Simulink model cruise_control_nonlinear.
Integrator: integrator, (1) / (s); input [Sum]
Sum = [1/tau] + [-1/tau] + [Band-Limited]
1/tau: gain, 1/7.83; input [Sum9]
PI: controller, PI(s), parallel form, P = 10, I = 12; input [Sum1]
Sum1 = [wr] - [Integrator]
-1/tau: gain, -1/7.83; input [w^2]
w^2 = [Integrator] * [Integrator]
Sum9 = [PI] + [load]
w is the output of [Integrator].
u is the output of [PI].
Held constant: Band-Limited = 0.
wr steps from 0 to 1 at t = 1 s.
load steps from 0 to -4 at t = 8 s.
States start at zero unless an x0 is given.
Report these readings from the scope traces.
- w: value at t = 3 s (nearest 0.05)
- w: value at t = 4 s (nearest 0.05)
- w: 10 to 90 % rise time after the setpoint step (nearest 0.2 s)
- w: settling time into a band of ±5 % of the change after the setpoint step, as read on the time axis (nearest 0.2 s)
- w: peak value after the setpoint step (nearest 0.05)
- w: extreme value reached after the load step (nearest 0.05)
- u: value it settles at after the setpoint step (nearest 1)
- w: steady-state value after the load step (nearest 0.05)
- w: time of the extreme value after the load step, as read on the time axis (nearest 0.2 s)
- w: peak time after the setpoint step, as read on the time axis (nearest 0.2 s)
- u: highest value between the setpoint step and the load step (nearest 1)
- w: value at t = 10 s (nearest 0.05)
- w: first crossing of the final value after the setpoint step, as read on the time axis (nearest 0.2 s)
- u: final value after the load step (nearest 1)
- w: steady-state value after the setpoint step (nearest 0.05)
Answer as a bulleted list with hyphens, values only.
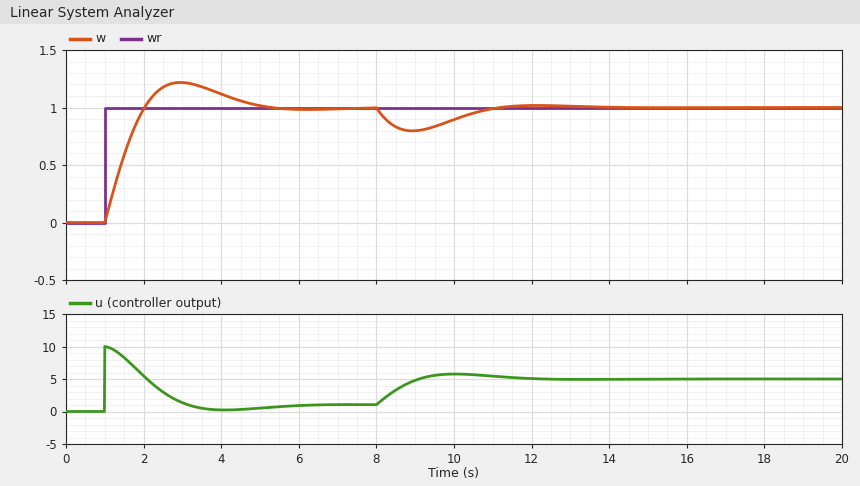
- 1.20
- 1.10
- 0.8 s
- 4.6 s
- 1.20
- 0.80
- 1
- 1.00
- 9.0 s
- 3.0 s
- 10
- 0.90
- 2.0 s
- 5
- 1.00
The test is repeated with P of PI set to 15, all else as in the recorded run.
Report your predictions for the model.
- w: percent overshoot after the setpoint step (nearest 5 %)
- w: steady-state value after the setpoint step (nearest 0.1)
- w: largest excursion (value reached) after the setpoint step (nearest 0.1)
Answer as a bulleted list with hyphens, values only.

- 15 %
- 1.0
- 1.1
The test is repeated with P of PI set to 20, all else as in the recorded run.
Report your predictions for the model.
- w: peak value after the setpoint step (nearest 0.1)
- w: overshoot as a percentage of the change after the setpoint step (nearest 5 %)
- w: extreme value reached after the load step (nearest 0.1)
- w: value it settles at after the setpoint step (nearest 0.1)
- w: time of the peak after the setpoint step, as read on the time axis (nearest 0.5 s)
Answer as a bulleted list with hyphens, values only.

- 1.1
- 10 %
- 0.9
- 1.0
- 2.5 s
